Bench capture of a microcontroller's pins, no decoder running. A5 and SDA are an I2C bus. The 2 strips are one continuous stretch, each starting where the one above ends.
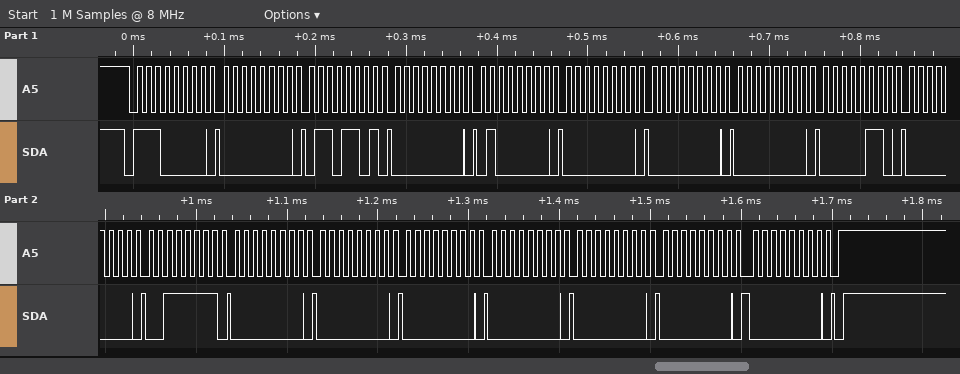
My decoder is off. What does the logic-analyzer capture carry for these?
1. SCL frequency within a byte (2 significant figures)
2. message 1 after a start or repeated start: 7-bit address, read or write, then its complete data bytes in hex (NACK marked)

100 kHz
0x70 write: 00 6D 00 40 00 00 00 06 00 3F 00 00 00 00 00 00 00
